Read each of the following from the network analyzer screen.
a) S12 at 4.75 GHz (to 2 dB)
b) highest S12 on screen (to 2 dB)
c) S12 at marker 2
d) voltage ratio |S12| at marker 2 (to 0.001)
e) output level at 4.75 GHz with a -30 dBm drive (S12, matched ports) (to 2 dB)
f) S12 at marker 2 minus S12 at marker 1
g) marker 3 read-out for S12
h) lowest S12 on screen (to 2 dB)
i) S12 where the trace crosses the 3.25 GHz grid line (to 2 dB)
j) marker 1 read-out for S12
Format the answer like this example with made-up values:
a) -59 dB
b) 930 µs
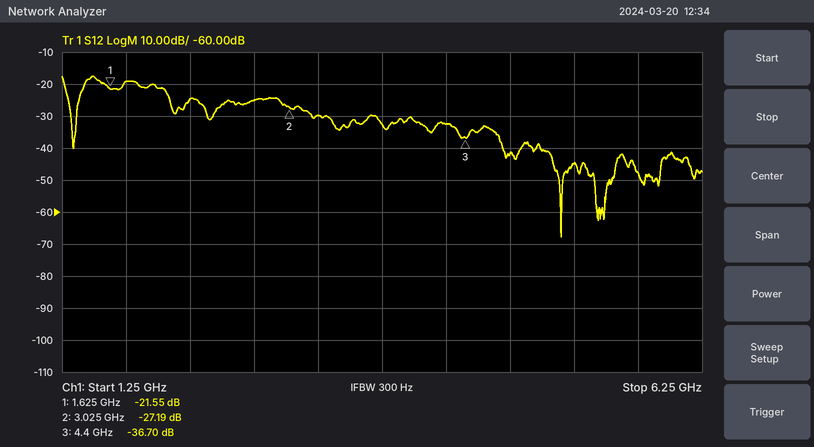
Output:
a) -42 dB
b) -18 dB
c) -27.19 dB
d) 0.044
e) -72 dBm
f) -5.64 dB
g) -36.70 dB
h) -68 dB
i) -30 dB
j) -21.55 dB
